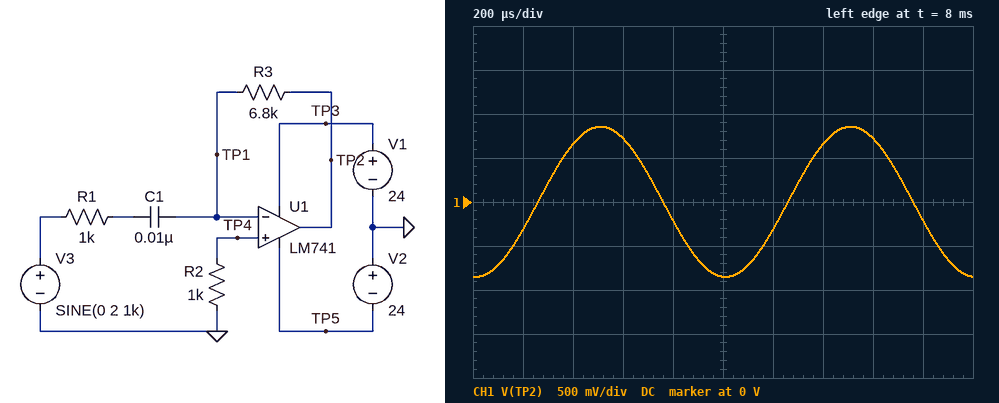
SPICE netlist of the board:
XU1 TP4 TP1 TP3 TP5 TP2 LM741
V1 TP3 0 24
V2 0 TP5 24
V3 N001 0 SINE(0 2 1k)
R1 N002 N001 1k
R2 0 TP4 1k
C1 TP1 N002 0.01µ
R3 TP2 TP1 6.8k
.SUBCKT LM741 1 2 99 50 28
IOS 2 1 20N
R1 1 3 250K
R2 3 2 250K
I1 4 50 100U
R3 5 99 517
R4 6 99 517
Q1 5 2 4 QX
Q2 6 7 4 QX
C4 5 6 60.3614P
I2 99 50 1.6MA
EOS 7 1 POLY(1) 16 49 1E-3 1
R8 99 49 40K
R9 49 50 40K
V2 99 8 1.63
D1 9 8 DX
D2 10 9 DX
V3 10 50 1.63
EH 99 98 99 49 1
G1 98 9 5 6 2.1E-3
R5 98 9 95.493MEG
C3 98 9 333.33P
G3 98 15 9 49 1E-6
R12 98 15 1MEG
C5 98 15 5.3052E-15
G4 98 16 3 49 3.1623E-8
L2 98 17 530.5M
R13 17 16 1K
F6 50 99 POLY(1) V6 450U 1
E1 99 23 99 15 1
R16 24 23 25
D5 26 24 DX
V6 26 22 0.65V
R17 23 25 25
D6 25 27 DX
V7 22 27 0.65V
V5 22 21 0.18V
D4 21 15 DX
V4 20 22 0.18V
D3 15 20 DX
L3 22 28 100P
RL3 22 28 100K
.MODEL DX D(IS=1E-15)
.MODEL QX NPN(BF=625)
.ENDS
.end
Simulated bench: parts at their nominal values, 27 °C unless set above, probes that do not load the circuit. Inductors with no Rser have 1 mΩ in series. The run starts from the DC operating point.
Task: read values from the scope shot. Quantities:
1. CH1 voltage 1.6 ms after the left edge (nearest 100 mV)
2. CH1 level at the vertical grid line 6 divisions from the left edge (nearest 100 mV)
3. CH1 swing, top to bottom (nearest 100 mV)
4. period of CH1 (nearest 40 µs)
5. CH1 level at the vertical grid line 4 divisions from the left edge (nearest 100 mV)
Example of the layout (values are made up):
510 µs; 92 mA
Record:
700 mV; -300 mV; 1.7 V; 1.00 ms; -200 mV
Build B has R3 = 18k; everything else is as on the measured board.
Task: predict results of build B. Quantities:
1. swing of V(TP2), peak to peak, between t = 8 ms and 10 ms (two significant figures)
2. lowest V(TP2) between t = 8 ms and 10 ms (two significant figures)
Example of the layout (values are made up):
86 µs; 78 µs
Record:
4.5 V; -2.3 V
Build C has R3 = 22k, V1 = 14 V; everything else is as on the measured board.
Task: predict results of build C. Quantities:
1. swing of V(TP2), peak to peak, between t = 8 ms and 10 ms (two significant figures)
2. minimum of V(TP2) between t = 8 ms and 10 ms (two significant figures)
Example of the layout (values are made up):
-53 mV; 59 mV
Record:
5.5 V; -2.8 V
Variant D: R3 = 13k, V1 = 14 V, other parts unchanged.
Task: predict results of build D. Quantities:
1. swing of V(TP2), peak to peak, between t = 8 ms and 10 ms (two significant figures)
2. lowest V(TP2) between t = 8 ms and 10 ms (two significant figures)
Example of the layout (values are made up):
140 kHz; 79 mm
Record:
3.3 V; -1.6 V
